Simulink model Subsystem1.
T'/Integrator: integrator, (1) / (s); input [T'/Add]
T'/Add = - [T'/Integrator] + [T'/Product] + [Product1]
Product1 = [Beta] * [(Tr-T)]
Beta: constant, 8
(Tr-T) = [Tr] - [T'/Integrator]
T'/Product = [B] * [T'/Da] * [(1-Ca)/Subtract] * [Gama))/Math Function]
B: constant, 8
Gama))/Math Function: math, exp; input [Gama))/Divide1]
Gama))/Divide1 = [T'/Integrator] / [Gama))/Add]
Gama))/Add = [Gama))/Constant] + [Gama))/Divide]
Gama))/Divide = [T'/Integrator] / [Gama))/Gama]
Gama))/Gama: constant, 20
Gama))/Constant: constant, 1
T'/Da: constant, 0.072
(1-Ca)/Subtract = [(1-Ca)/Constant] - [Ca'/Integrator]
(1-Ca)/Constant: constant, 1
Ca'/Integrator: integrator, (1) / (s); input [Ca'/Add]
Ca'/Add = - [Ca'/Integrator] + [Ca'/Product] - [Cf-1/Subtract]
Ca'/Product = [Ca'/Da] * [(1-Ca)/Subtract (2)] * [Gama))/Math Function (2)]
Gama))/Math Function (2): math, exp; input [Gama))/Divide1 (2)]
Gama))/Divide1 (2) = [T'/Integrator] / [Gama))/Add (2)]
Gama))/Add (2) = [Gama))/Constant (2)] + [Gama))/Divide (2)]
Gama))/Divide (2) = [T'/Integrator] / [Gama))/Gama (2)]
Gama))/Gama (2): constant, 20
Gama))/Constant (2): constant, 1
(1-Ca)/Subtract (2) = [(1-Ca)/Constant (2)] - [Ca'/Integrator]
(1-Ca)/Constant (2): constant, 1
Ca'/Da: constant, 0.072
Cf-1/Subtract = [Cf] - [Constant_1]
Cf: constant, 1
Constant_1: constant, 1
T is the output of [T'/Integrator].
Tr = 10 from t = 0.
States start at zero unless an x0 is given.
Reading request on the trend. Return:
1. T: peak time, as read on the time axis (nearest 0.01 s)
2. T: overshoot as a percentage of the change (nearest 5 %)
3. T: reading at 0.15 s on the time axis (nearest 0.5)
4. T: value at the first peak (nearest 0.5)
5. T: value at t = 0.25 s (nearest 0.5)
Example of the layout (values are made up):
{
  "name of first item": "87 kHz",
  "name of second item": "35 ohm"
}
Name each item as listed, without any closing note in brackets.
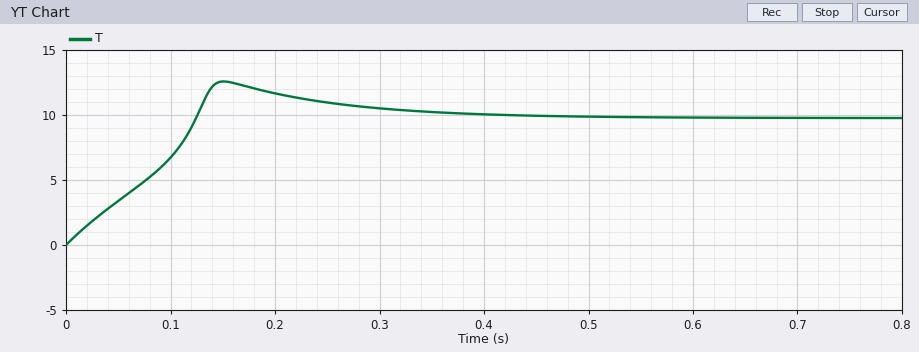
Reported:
{
  "T: peak time, as read on the time axis": "0.15 s",
  "T: overshoot as a percentage of the change": "30 %",
  "T: reading at 0.15 s on the time axis": "12.5",
  "T: value at the first peak": "12.5",
  "T: value at t = 0.25 s": "11.0"
}
